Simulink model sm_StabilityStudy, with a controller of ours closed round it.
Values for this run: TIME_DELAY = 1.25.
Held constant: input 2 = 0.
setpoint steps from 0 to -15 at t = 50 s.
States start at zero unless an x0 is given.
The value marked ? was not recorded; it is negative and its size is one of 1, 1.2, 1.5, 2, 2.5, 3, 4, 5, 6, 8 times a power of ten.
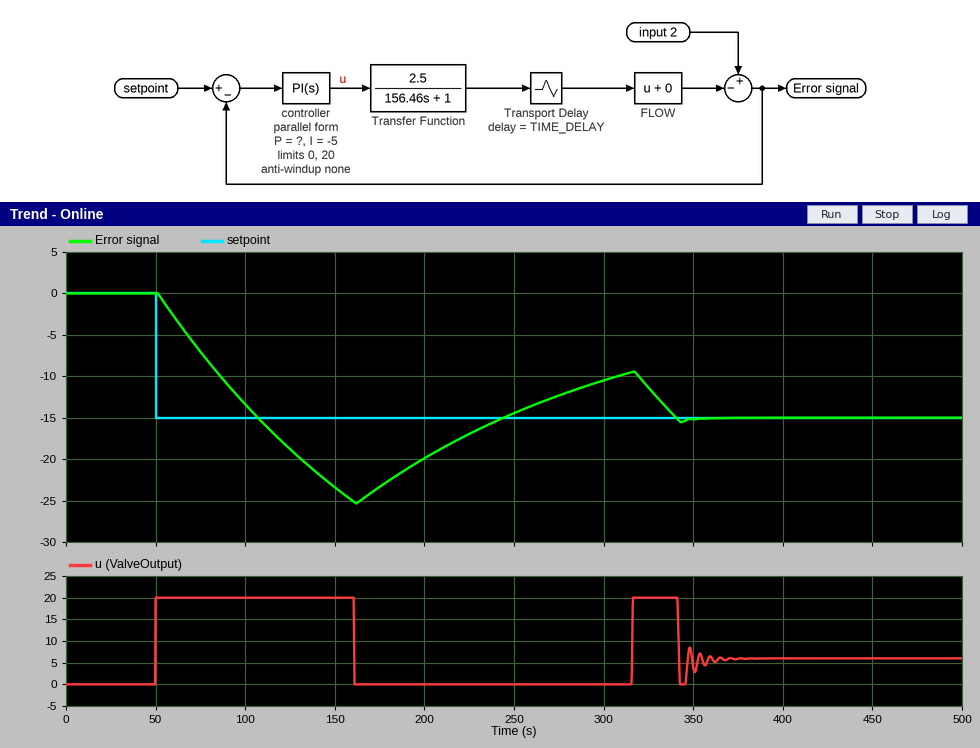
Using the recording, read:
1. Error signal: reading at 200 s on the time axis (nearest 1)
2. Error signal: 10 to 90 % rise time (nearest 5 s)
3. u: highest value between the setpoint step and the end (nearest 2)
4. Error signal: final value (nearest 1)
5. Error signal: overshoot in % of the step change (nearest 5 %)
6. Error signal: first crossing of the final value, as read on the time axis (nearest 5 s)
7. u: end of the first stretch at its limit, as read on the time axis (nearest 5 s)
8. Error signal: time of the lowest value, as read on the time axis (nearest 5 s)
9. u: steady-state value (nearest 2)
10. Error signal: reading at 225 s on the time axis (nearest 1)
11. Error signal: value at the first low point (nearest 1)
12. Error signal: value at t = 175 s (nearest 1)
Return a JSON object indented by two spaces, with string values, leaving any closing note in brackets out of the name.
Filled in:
{
  "Error signal: reading at 200 s on the time axis": "-20",
  "Error signal: 10 to 90 % rise time": "45 s",
  "u: highest value between the setpoint step and the end": "20",
  "Error signal: final value": "-15",
  "Error signal: overshoot in % of the step change": "70 %",
  "Error signal: first crossing of the final value, as read on the time axis": "105 s",
  "u: end of the first stretch at its limit, as read on the time axis": "160 s",
  "Error signal: time of the lowest value, as read on the time axis": "160 s",
  "u: steady-state value": "6",
  "Error signal: reading at 225 s on the time axis": "-17",
  "Error signal: value at the first low point": "-25",
  "Error signal: value at t = 175 s": "-23"
}
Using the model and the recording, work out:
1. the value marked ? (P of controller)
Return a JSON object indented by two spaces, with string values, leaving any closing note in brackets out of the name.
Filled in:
{
  "the value marked ?": "-60"
}
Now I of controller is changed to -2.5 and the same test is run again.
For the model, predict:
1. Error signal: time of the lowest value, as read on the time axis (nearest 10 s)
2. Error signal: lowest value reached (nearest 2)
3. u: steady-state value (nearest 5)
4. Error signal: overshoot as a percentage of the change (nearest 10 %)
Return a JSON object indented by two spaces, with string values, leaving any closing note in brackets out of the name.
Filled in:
{
  "Error signal: time of the lowest value, as read on the time axis": "150 s",
  "Error signal: lowest value reached": "-24",
  "u: steady-state value": "5",
  "Error signal: overshoot as a percentage of the change": "60 %"
}
